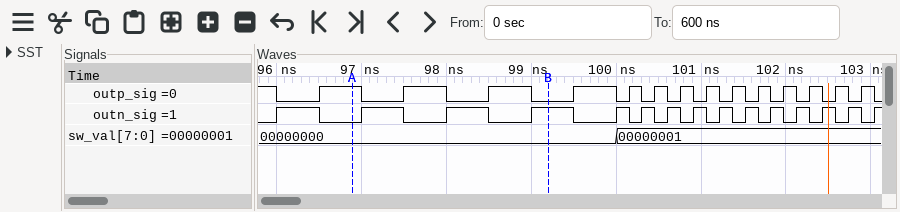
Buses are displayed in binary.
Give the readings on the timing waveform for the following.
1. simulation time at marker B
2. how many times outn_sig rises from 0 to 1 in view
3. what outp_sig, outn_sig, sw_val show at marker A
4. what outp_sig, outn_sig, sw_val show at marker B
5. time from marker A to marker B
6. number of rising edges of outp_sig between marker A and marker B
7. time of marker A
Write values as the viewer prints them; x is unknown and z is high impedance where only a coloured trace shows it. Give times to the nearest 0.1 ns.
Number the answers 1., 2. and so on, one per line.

1. 99.2 ns
2. 15
3. outp_sig=1, outn_sig=0, sw_val=00000000
4. outp_sig=0, outn_sig=1, sw_val=00000000
5. 2.3 ns
6. 2
7. 96.9 ns
